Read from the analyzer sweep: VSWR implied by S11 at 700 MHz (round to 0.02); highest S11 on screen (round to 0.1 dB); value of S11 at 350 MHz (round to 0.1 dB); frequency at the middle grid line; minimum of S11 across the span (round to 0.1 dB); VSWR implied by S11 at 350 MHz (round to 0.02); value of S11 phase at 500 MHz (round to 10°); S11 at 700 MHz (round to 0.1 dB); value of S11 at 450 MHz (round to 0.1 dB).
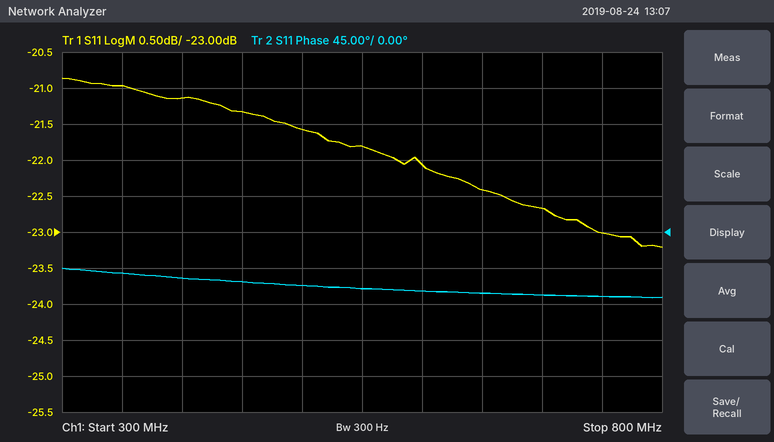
1.16
-20.9 dB
-21.0 dB
550 MHz
-23.2 dB
1.20
-70°
-22.7 dB
-21.3 dB
